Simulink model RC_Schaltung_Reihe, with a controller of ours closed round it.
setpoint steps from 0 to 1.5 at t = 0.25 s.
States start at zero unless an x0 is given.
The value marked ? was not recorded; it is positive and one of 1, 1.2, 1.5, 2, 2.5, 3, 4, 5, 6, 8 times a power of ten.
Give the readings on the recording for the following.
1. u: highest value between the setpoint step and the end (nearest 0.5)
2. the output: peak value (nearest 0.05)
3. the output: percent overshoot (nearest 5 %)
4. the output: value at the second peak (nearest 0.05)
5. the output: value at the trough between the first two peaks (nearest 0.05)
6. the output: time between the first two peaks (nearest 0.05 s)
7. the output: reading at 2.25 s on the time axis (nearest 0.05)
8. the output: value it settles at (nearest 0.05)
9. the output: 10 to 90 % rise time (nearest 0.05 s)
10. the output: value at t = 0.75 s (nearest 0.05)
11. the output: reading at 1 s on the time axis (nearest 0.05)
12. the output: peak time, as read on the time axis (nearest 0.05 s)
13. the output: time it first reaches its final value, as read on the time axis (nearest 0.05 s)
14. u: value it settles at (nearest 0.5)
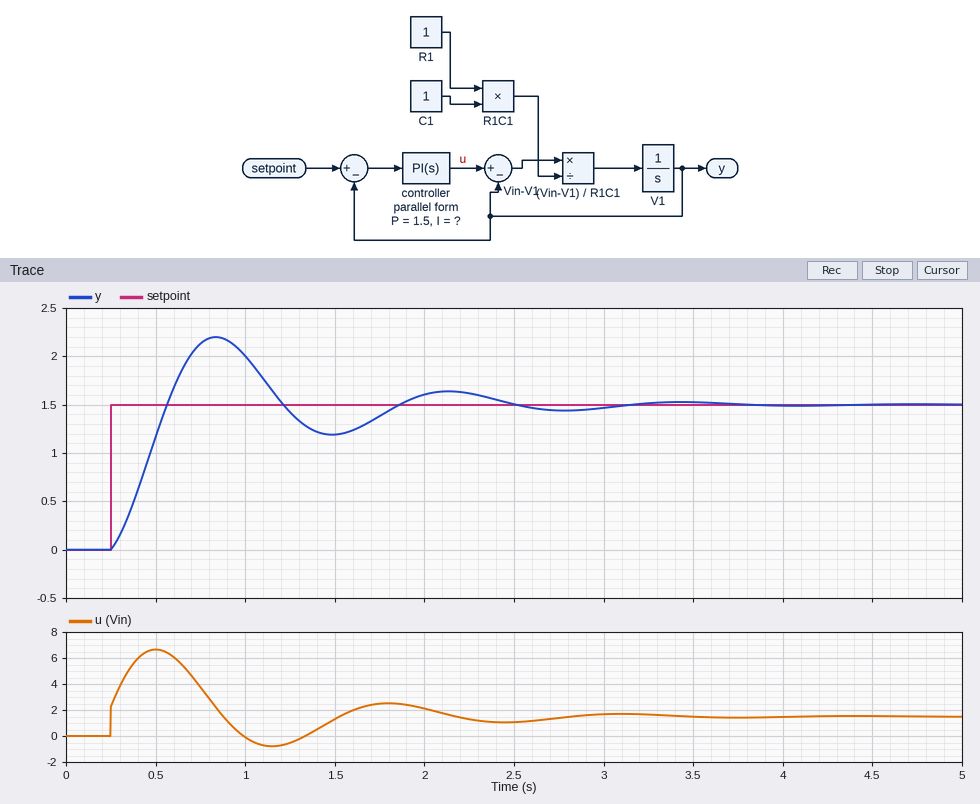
6.5
2.20
45 %
1.65
1.20
1.30 s
1.60
1.50
0.25 s
2.15
2.00
0.85 s
0.55 s
1.5
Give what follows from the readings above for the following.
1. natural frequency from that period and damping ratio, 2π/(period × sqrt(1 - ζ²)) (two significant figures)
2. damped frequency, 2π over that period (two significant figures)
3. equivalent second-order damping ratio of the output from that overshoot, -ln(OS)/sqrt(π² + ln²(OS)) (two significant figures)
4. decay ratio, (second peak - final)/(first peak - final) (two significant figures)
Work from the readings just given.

5.0 rad/s
4.8 rad/s
0.25
0.21
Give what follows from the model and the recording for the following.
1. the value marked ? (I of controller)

25
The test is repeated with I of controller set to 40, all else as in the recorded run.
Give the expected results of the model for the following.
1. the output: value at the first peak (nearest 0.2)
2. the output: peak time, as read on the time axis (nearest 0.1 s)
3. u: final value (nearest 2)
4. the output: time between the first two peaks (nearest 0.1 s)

2.4
0.7 s
2
1.0 s
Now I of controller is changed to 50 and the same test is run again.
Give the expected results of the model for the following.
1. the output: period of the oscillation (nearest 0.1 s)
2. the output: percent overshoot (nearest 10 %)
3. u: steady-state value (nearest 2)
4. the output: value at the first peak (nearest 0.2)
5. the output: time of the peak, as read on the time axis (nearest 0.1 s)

0.9 s
60 %
2
2.4
0.7 s
